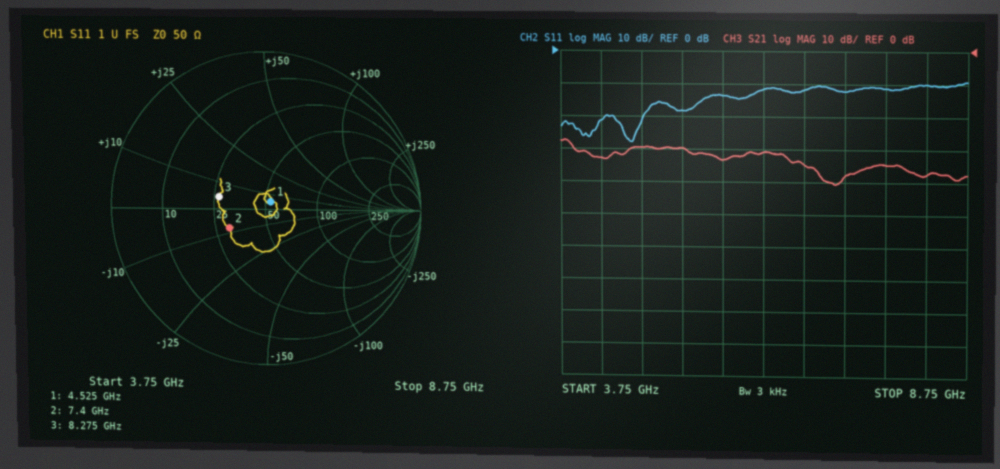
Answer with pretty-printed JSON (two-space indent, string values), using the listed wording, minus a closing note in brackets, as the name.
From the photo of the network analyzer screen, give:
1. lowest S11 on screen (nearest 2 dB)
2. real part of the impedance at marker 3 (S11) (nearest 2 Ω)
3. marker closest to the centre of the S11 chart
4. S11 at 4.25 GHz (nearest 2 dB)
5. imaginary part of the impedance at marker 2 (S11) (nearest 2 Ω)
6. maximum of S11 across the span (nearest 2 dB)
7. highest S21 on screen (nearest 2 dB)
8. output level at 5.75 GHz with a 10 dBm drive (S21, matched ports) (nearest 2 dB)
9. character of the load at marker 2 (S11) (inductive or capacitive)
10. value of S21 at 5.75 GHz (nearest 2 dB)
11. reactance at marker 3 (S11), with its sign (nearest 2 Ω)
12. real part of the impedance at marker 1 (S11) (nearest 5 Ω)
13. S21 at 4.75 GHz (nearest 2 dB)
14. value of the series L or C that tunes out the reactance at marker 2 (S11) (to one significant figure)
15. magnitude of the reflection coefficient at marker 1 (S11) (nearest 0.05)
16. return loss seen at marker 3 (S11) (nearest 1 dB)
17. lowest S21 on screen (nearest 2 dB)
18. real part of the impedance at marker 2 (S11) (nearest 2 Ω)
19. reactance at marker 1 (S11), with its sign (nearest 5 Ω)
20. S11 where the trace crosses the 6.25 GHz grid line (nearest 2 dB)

{
  "lowest S11 on screen": "-28 dB",
  "real part of the impedance at marker 3 (S11)": "26 Ω",
  "marker closest to the centre of the S11 chart": "marker 1",
  "S11 at 4.25 GHz": "-22 dB",
  "imaginary part of the impedance at marker 2 (S11)": "-8 Ω",
  "maximum of S11 across the span": "-10 dB",
  "highest S21 on screen": "-28 dB",
  "output level at 5.75 GHz with a 10 dBm drive (S21, matched ports)": "-24 dBm",
  "character of the load at marker 2 (S11)": "capacitive",
  "value of S21 at 5.75 GHz": "-34 dB",
  "reactance at marker 3 (S11), with its sign": "+4 Ω",
  "real part of the impedance at marker 1 (S11)": "55 Ω",
  "S21 at 4.75 GHz": "-30 dB",
  "value of the series L or C that tunes out the reactance at marker 2 (S11)": "200 pH",
  "magnitude of the reflection coefficient at marker 1 (S11)": "0.05",
  "return loss seen at marker 3 (S11)": "10 dB",
  "lowest S21 on screen": "-40 dB",
  "real part of the impedance at marker 2 (S11)": "30 Ω",
  "reactance at marker 1 (S11), with its sign": "+5 Ω",
  "S11 where the trace crosses the 6.25 GHz grid line": "-12 dB"
}
